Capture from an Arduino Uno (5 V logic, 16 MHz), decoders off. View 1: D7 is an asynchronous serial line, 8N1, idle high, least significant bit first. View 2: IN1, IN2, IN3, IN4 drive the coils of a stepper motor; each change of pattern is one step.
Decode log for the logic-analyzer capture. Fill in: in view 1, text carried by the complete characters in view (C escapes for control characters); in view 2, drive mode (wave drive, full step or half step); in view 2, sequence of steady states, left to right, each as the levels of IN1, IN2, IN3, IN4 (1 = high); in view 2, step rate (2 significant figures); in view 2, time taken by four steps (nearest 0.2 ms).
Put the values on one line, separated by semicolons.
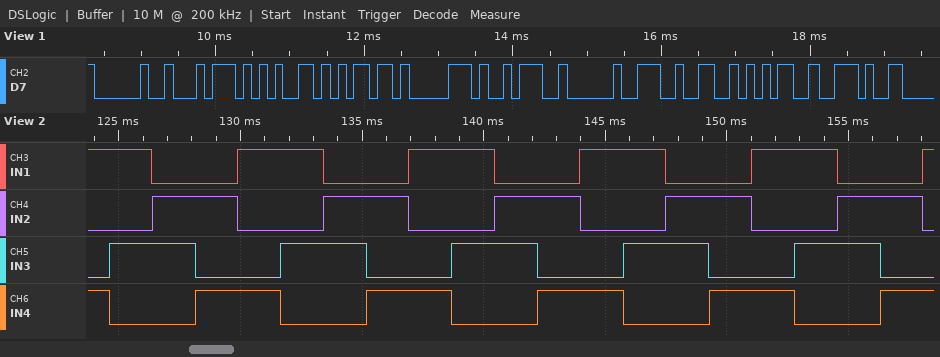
" temp: 25."; full step; 1001 1010 0110 0101 1001 1010 0110 0101 1001 1010 0110 0101 1001 1010 0110 0101 1001 1010 0110 0101 1001; 570 steps/s; 7.0 ms
